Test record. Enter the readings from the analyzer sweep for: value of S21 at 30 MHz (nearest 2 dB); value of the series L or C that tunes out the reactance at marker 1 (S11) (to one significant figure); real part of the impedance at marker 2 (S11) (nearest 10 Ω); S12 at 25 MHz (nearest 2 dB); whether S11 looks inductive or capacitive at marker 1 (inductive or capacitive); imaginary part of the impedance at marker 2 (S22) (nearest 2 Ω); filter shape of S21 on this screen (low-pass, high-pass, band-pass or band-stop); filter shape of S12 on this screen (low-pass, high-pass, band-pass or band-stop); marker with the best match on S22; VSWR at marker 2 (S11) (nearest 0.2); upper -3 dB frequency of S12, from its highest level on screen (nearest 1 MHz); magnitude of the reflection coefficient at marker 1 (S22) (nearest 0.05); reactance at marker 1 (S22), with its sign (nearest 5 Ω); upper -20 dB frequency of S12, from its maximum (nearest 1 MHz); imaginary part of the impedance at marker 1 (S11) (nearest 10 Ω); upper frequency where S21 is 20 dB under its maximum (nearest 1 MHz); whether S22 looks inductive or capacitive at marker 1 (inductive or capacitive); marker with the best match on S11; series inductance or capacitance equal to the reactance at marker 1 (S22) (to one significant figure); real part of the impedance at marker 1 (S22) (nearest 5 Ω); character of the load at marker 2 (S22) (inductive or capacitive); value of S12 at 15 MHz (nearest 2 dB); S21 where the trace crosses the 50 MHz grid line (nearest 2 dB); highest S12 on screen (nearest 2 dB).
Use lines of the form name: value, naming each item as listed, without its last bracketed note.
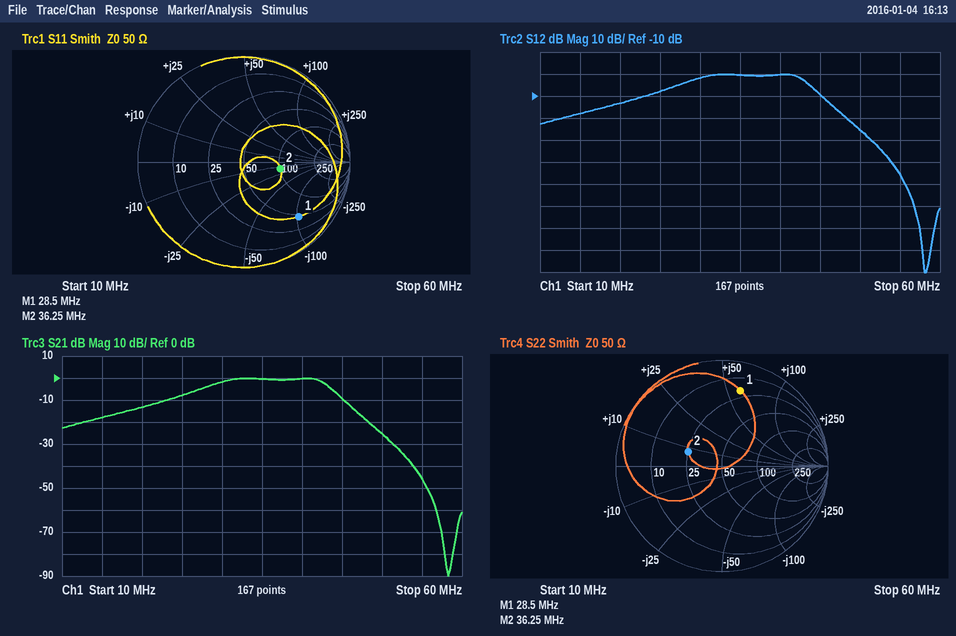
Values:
value of S21 at 30 MHz: -2 dB
value of the series L or C that tunes out the reactance at marker 1 (S11): 600 nH
real part of the impedance at marker 2 (S11): 100 Ω
S12 at 25 MHz: -8 dB
whether S11 looks inductive or capacitive at marker 1: capacitive
imaginary part of the impedance at marker 2 (S22): +8 Ω
filter shape of S21 on this screen: band-pass
filter shape of S12 on this screen: band-pass
marker with the best match on S22: marker 2
VSWR at marker 2 (S11): 2.0
upper -3 dB frequency of S12, from its highest level on screen: 43 MHz
magnitude of the reflection coefficient at marker 1 (S22): 0.75
reactance at marker 1 (S22), with its sign: +60 Ω
upper -20 dB frequency of S12, from its maximum: 48 MHz
imaginary part of the impedance at marker 1 (S11): -100 Ω
upper frequency where S21 is 20 dB under its maximum: 48 MHz
whether S22 looks inductive or capacitive at marker 1: inductive
marker with the best match on S11: marker 2
series inductance or capacitance equal to the reactance at marker 1 (S22): 300 nH
real part of the impedance at marker 1 (S22): 20 Ω
character of the load at marker 2 (S22): inductive
value of S12 at 15 MHz: -18 dB
S21 where the trace crosses the 50 MHz grid line: -26 dB
highest S12 on screen: 0 dB
